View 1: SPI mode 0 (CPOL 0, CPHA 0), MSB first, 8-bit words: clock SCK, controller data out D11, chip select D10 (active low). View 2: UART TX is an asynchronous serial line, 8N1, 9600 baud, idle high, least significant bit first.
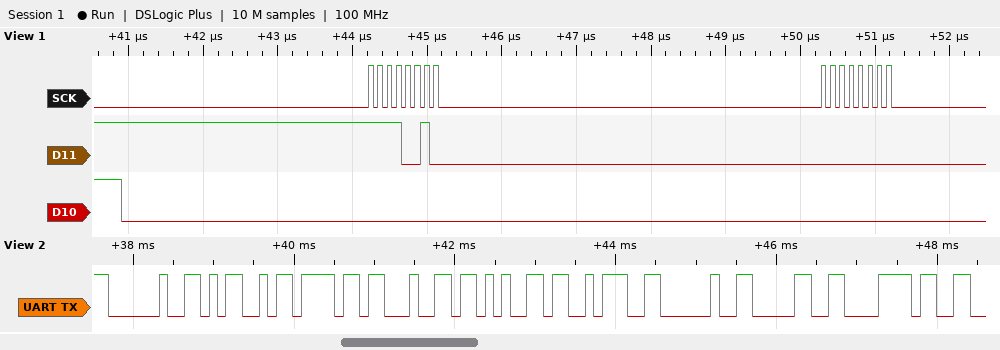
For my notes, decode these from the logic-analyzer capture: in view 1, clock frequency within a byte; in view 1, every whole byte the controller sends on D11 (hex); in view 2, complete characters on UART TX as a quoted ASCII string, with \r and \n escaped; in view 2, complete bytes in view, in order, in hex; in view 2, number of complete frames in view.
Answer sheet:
8 MHz
F2 00
" Mode: 0x"
20 4D 6F 64 65 3A 20 30 78
9
